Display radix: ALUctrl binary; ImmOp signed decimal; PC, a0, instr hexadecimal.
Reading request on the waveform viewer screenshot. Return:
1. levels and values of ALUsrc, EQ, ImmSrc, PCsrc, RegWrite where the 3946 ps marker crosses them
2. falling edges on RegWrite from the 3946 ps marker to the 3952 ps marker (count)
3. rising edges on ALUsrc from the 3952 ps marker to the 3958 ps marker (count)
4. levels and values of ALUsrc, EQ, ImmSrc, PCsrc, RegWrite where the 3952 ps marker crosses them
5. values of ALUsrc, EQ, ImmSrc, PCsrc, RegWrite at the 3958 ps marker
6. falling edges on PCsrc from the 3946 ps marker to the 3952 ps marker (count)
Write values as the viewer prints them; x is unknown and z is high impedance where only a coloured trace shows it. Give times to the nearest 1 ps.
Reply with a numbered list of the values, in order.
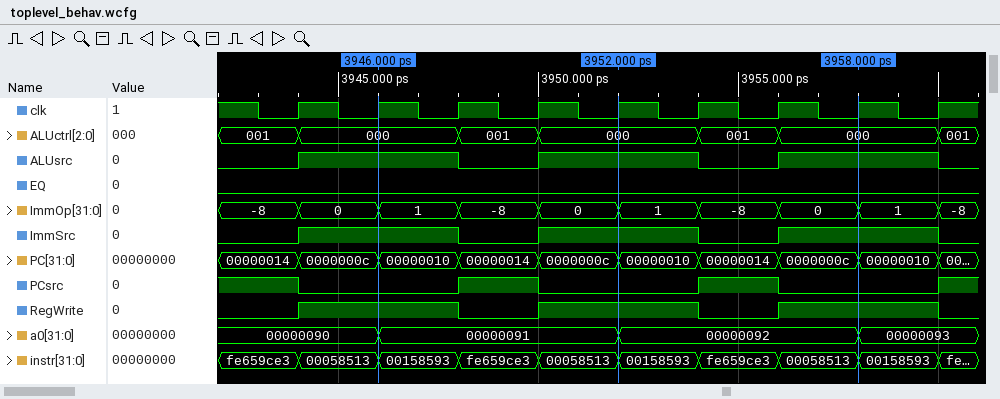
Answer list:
1. ALUsrc=1, EQ=0, ImmSrc=1, PCsrc=0, RegWrite=1
2. 1
3. 1
4. ALUsrc=1, EQ=0, ImmSrc=1, PCsrc=0, RegWrite=1
5. ALUsrc=1, EQ=0, ImmSrc=1, PCsrc=0, RegWrite=1
6. 1
